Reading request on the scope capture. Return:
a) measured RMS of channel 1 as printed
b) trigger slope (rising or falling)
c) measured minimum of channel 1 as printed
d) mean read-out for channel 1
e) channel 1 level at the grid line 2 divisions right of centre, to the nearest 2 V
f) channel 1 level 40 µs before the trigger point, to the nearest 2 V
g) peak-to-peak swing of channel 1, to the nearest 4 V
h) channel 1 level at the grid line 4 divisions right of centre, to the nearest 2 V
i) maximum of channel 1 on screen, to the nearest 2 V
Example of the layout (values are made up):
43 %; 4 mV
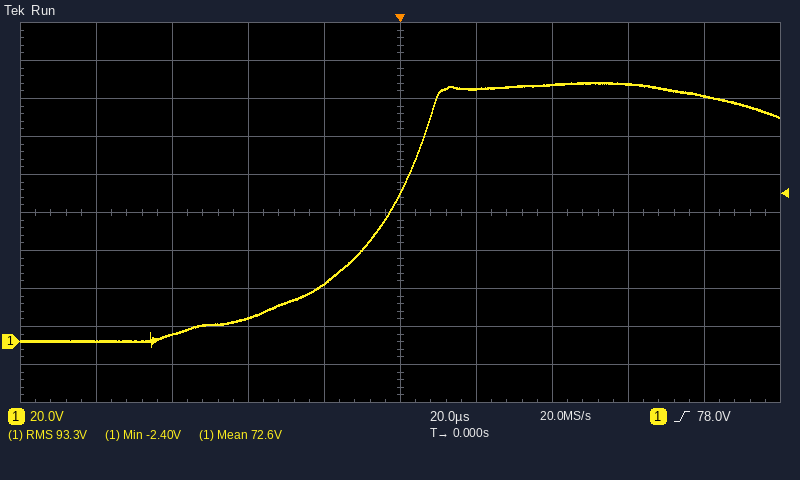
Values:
93.3 V; rising; -2.40 V; 72.6 V; 136 V; 12 V; 140 V; 130 V; 136 V
